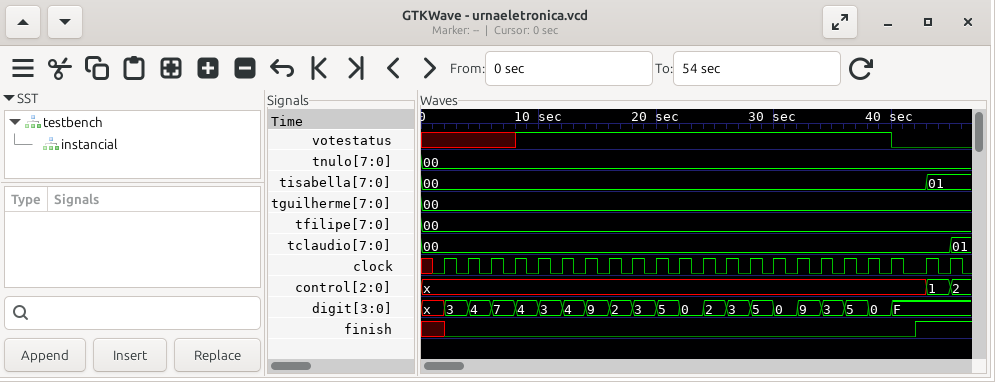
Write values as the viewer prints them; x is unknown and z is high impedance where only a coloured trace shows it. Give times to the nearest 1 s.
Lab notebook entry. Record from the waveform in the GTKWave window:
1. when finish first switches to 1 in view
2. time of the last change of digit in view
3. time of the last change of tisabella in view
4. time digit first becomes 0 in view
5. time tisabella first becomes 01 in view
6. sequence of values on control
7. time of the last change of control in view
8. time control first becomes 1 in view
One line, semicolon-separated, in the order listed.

42 s; 40 s; 43 s; 22 s; 43 s; x, 1, 2; 45 s; 43 s
